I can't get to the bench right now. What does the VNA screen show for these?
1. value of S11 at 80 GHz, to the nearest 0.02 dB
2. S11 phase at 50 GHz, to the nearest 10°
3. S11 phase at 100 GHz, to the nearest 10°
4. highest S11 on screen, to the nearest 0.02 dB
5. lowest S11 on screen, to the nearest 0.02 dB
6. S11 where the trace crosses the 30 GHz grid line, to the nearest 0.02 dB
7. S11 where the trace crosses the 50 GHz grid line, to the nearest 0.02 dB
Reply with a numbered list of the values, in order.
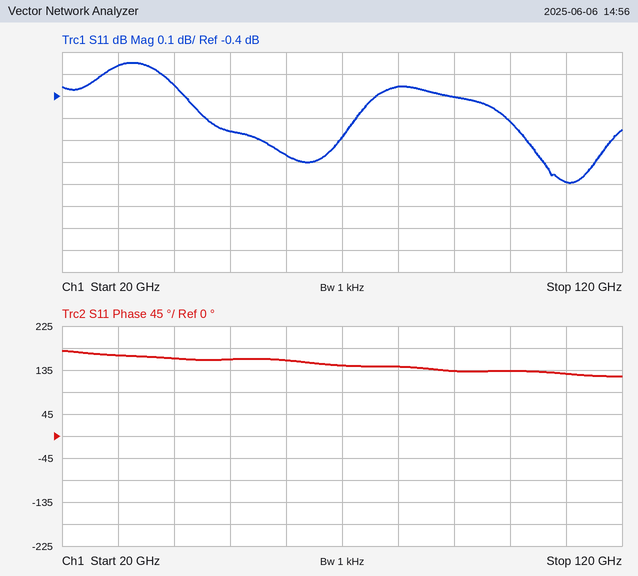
1. -0.36 dB
2. 160°
3. 130°
4. -0.24 dB
5. -0.80 dB
6. -0.26 dB
7. -0.56 dB
